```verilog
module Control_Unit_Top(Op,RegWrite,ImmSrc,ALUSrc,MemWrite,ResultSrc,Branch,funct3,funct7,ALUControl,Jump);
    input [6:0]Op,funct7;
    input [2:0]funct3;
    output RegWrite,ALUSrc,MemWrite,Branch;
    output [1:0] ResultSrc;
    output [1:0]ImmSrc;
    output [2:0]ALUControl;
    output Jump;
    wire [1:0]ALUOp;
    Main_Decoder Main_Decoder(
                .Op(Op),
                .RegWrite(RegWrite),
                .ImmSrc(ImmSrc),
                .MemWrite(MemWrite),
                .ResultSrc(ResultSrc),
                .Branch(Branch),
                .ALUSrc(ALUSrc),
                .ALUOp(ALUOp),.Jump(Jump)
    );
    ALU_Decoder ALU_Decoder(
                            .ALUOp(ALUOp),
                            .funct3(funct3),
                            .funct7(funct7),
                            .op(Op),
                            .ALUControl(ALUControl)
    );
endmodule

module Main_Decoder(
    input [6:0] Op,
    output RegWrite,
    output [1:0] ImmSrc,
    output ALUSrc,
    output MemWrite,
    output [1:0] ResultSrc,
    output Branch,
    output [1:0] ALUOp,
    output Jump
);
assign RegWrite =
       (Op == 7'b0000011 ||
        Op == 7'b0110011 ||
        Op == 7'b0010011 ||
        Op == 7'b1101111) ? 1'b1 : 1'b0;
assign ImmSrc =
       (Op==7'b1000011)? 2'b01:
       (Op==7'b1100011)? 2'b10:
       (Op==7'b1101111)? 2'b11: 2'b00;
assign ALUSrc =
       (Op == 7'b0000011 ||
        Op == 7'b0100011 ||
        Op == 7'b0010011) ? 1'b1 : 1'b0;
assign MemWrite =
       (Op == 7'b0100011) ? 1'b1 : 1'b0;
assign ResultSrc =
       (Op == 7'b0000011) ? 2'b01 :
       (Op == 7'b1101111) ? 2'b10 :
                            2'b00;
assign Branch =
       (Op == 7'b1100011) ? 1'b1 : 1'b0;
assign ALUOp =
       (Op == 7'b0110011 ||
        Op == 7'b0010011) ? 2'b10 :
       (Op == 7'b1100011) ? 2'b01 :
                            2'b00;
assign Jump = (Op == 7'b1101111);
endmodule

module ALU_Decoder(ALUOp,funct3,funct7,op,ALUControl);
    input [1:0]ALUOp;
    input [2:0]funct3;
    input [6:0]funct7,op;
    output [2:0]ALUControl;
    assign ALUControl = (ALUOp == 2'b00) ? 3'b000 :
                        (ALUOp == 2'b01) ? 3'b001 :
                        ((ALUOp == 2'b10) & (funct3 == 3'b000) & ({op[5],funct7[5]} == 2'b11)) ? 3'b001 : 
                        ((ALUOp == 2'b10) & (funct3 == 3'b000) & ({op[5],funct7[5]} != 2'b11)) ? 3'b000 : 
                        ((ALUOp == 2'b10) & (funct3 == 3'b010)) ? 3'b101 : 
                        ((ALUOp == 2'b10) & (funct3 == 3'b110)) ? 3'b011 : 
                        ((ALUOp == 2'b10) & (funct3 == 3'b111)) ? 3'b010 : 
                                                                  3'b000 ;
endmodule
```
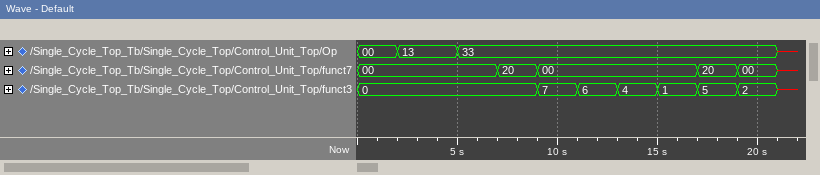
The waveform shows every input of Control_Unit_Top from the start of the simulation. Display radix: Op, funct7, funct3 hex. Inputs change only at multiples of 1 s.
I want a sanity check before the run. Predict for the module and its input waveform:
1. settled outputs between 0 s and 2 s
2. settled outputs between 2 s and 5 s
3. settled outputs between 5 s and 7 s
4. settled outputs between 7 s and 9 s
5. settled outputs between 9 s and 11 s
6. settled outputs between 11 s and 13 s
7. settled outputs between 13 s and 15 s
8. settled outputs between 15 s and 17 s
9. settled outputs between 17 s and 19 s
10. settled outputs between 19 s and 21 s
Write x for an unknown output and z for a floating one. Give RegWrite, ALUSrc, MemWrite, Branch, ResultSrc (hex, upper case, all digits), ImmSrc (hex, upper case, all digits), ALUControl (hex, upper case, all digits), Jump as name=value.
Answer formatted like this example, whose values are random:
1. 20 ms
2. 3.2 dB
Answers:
1. RegWrite=0, ALUSrc=0, MemWrite=0, Branch=0, ResultSrc=0, ImmSrc=0, ALUControl=0, Jump=0
2. RegWrite=1, ALUSrc=1, MemWrite=0, Branch=0, ResultSrc=0, ImmSrc=0, ALUControl=0, Jump=0
3. RegWrite=1, ALUSrc=0, MemWrite=0, Branch=0, ResultSrc=0, ImmSrc=0, ALUControl=0, Jump=0
4. RegWrite=1, ALUSrc=0, MemWrite=0, Branch=0, ResultSrc=0, ImmSrc=0, ALUControl=1, Jump=0
5. RegWrite=1, ALUSrc=0, MemWrite=0, Branch=0, ResultSrc=0, ImmSrc=0, ALUControl=2, Jump=0
6. RegWrite=1, ALUSrc=0, MemWrite=0, Branch=0, ResultSrc=0, ImmSrc=0, ALUControl=3, Jump=0
7. RegWrite=1, ALUSrc=0, MemWrite=0, Branch=0, ResultSrc=0, ImmSrc=0, ALUControl=0, Jump=0
8. RegWrite=1, ALUSrc=0, MemWrite=0, Branch=0, ResultSrc=0, ImmSrc=0, ALUControl=0, Jump=0
9. RegWrite=1, ALUSrc=0, MemWrite=0, Branch=0, ResultSrc=0, ImmSrc=0, ALUControl=0, Jump=0
10. RegWrite=1, ALUSrc=0, MemWrite=0, Branch=0, ResultSrc=0, ImmSrc=0, ALUControl=5, Jump=0
